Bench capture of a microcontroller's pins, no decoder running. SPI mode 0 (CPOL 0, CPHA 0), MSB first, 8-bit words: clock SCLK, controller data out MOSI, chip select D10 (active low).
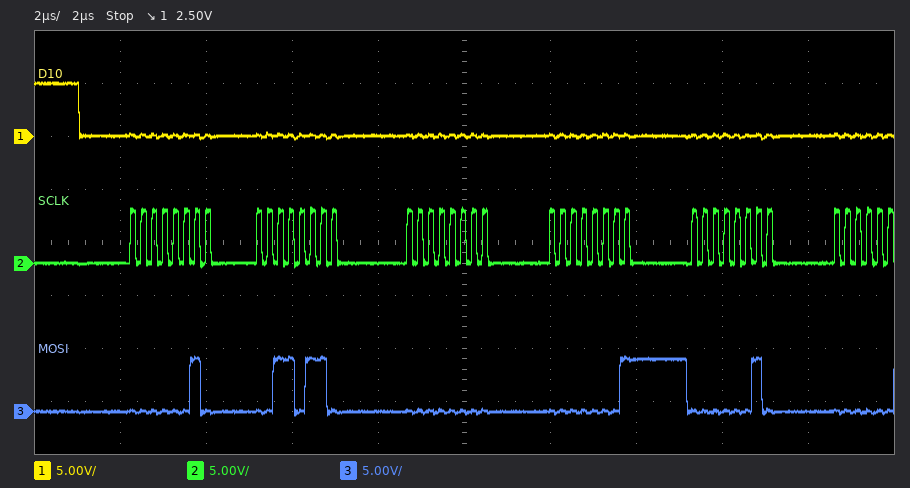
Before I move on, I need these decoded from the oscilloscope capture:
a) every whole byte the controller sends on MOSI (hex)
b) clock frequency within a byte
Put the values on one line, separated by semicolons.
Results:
02 36 00 01 02; 4 MHz
